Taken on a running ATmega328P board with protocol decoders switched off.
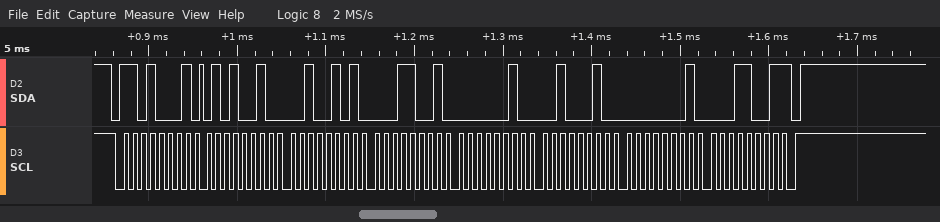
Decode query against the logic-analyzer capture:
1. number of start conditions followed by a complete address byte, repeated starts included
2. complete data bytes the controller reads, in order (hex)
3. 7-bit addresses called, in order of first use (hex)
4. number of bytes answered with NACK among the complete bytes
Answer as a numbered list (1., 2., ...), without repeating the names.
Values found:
1. 1
2. 52 25 19 02 22 01 19
3. 0x68
4. 1
